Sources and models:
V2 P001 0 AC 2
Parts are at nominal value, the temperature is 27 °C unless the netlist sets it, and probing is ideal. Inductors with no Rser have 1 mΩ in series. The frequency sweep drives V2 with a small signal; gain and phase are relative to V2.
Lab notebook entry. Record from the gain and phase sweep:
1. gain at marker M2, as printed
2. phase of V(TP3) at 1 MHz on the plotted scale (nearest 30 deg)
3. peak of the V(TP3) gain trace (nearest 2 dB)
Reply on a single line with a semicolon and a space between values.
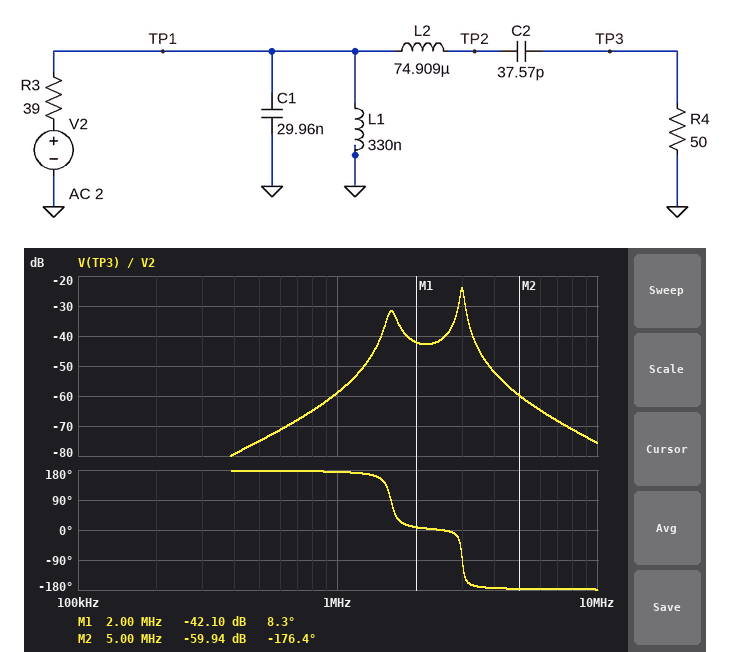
-59.94 dB; 180 deg; -24 dB
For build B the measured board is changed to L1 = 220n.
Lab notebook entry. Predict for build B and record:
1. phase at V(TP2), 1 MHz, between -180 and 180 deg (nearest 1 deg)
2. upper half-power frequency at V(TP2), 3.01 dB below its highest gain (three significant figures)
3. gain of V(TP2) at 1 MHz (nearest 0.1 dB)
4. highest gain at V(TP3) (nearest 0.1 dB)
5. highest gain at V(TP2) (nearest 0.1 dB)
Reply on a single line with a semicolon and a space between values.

87 deg; 3.05 MHz; -25.4 dB; -22.1 dB; 6.9 dB
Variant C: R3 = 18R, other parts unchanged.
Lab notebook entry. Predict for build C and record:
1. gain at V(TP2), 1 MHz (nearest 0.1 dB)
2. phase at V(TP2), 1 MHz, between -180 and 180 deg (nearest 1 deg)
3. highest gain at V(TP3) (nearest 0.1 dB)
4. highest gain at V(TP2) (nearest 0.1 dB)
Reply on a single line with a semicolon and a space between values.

-13.6 dB; 79 deg; -17.4 dB; 11.6 dB
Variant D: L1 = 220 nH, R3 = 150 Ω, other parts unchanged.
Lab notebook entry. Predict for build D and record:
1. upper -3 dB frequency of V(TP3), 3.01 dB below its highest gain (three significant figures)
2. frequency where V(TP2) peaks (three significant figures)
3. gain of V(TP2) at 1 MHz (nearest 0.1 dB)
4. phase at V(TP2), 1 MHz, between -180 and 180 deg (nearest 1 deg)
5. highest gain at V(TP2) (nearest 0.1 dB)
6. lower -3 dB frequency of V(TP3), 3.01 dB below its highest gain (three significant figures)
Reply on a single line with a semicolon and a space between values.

1.98 MHz; 1.96 MHz; -37.1 dB; 89 deg; 4.6 dB; 1.94 MHz
